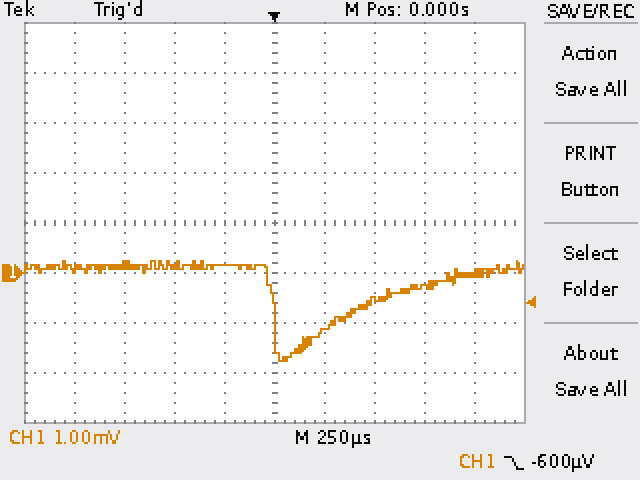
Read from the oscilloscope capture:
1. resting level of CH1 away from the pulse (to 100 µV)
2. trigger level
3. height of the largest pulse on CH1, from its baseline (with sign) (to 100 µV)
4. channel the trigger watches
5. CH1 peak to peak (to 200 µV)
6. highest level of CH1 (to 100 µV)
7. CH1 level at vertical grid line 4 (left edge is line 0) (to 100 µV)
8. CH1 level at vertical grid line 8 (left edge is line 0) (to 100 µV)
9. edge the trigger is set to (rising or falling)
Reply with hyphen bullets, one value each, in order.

- 100 µV
- -600 µV
- -1.9 mV
- CH1
- 2.0 mV
- 200 µV
- 200 µV
- -300 µV
- falling
